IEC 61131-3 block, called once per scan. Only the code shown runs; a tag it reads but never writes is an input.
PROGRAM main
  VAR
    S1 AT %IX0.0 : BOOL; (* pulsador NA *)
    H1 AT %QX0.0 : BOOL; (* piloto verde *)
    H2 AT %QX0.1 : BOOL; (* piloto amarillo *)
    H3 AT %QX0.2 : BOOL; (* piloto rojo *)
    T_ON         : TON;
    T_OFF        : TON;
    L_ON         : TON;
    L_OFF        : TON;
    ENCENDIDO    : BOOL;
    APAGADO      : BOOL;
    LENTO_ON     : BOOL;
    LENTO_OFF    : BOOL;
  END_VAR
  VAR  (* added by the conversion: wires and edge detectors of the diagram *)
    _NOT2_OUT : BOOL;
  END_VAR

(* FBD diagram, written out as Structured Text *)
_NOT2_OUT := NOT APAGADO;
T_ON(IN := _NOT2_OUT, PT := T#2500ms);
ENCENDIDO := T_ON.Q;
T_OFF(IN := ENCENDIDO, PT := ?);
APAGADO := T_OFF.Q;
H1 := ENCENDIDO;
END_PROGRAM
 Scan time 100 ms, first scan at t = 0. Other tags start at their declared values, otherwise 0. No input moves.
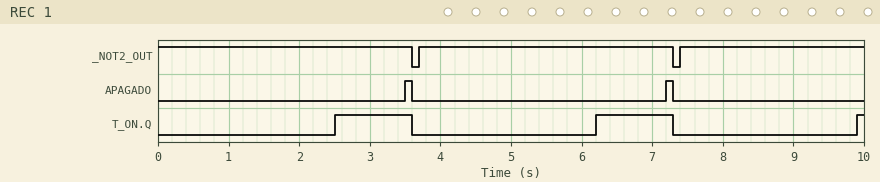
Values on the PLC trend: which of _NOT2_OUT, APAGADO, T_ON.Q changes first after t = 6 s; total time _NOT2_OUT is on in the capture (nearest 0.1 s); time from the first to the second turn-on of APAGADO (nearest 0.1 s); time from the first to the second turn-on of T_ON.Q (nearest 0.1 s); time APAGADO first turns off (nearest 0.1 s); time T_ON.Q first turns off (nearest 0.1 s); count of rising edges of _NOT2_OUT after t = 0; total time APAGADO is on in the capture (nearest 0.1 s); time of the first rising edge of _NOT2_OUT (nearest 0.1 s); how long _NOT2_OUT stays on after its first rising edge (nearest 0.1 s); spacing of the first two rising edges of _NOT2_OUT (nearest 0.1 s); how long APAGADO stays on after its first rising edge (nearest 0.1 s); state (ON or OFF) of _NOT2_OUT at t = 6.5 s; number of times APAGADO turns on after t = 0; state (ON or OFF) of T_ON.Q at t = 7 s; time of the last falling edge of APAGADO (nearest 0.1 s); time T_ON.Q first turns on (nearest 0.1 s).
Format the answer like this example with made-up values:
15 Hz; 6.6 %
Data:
T_ON.Q; 9.8 s; 3.7 s; 3.7 s; 3.6 s; 3.6 s; 2; 0.2 s; 3.7 s; 3.6 s; 3.7 s; 0.1 s; ON; 2; ON; 7.3 s; 2.5 s
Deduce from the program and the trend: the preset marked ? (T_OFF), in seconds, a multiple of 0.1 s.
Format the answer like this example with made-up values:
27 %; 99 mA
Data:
1.0 s
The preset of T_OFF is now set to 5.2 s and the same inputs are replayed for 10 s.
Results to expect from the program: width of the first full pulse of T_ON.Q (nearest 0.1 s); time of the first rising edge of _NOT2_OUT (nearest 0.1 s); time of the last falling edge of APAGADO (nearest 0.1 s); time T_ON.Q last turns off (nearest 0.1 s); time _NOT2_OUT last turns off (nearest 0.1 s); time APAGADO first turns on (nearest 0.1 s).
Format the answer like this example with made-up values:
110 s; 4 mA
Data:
5.3 s; 7.9 s; 7.8 s; 7.8 s; 7.8 s; 7.7 s
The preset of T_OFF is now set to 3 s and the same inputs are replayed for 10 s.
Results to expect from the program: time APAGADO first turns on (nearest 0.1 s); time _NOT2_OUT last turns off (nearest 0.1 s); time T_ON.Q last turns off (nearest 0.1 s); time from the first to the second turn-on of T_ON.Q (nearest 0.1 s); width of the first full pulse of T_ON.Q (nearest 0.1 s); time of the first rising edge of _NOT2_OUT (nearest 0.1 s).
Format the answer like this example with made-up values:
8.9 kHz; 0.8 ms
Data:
5.5 s; 5.6 s; 5.6 s; 5.7 s; 3.1 s; 5.7 s
